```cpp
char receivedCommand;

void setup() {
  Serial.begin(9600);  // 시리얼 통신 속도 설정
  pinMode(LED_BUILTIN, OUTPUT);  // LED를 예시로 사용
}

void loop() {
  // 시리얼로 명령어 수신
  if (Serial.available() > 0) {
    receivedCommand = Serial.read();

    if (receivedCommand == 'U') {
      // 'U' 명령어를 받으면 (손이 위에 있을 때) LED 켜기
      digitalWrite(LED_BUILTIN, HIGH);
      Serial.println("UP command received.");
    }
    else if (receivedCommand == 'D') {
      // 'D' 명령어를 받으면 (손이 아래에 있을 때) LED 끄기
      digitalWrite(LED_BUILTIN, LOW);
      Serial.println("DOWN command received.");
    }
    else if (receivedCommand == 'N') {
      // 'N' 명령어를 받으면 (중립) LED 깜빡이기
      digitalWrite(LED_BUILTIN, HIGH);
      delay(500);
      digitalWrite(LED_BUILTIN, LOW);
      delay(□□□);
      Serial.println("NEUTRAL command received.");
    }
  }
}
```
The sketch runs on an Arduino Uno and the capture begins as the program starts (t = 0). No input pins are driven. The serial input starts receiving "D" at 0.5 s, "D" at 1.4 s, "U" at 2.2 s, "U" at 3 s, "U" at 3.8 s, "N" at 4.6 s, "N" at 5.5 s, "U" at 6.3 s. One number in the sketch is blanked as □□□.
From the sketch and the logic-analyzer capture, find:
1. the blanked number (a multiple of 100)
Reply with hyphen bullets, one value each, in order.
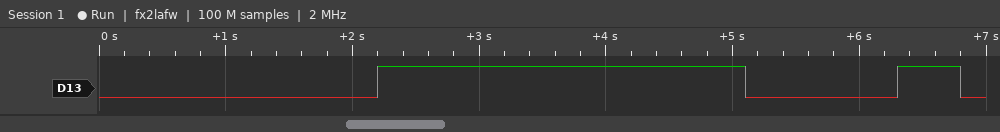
- 1200
